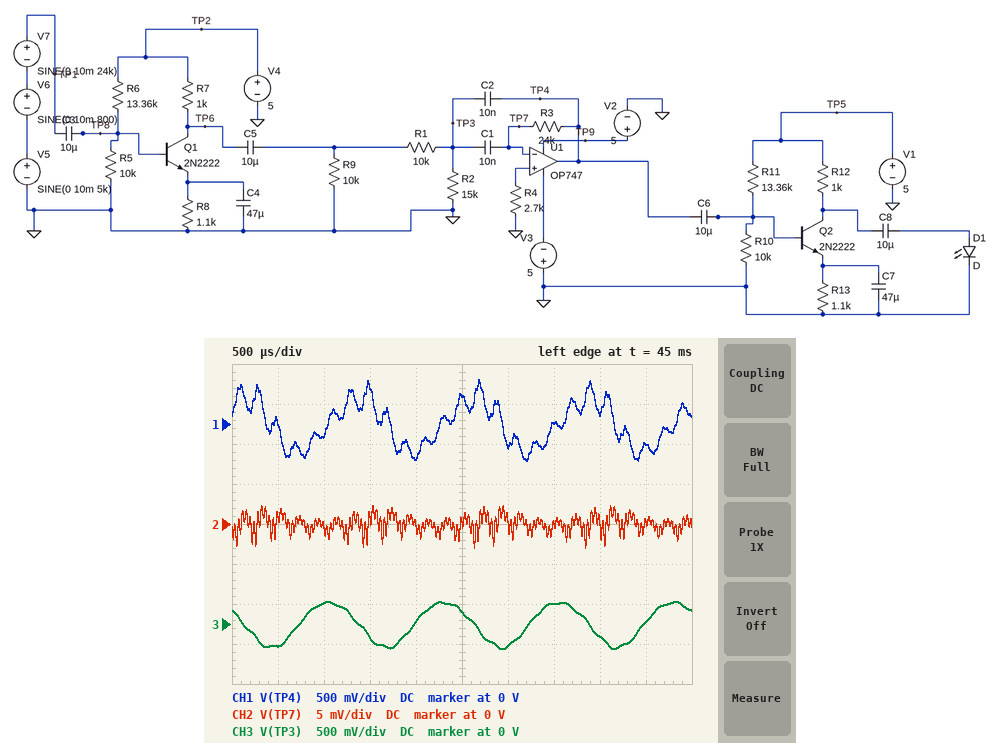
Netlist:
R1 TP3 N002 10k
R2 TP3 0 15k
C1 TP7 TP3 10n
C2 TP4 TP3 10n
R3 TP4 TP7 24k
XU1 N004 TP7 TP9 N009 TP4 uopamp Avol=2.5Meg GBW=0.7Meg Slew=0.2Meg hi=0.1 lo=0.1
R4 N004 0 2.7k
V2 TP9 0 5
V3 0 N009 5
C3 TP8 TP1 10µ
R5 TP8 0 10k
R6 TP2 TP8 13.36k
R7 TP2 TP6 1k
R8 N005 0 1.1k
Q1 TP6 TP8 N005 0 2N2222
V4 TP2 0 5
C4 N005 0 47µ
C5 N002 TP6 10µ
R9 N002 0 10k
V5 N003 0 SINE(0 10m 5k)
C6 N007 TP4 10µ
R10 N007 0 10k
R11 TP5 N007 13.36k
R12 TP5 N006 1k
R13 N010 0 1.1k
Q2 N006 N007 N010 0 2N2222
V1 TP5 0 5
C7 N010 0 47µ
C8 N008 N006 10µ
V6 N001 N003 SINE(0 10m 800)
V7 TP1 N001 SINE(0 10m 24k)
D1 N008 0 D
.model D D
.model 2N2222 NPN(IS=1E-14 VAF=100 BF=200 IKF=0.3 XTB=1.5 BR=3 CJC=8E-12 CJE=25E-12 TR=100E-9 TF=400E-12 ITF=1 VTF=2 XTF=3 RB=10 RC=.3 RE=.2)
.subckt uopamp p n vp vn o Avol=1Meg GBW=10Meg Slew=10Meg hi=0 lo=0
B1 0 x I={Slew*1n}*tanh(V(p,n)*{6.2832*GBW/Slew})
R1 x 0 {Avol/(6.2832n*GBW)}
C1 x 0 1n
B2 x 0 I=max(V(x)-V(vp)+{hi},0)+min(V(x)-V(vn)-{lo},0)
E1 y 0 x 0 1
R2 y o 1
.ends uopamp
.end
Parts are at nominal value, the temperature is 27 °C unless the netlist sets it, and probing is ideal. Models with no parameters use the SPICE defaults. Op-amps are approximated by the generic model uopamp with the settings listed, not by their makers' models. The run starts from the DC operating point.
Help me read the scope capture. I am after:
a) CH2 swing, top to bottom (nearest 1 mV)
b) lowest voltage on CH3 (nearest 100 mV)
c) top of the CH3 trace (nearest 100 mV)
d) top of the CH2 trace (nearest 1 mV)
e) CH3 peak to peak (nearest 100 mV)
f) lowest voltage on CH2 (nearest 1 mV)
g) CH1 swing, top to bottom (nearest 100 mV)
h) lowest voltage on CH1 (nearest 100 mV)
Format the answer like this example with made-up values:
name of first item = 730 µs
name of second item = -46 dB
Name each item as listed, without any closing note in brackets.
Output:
CH2 swing, top to bottom = 5 mV
lowest voltage on CH3 = -300 mV
top of the CH3 trace = 300 mV
top of the CH2 trace = 2 mV
CH3 peak to peak = 600 mV
lowest voltage on CH2 = -3 mV
CH1 swing, top to bottom = 1.0 V
lowest voltage on CH1 = -500 mV
